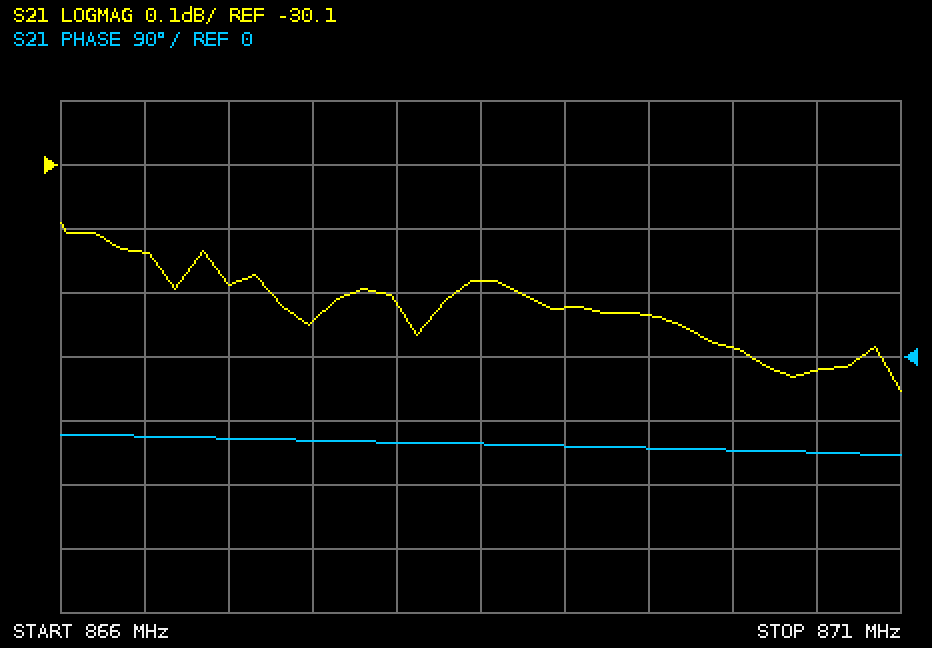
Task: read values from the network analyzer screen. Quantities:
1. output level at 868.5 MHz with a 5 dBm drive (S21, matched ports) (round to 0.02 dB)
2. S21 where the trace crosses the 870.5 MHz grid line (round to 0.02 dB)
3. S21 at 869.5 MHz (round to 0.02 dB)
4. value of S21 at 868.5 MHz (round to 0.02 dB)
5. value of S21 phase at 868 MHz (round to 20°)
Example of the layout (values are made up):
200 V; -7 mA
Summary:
-25.28 dBm; -30.42 dB; -30.34 dB; -30.28 dB; -120°
